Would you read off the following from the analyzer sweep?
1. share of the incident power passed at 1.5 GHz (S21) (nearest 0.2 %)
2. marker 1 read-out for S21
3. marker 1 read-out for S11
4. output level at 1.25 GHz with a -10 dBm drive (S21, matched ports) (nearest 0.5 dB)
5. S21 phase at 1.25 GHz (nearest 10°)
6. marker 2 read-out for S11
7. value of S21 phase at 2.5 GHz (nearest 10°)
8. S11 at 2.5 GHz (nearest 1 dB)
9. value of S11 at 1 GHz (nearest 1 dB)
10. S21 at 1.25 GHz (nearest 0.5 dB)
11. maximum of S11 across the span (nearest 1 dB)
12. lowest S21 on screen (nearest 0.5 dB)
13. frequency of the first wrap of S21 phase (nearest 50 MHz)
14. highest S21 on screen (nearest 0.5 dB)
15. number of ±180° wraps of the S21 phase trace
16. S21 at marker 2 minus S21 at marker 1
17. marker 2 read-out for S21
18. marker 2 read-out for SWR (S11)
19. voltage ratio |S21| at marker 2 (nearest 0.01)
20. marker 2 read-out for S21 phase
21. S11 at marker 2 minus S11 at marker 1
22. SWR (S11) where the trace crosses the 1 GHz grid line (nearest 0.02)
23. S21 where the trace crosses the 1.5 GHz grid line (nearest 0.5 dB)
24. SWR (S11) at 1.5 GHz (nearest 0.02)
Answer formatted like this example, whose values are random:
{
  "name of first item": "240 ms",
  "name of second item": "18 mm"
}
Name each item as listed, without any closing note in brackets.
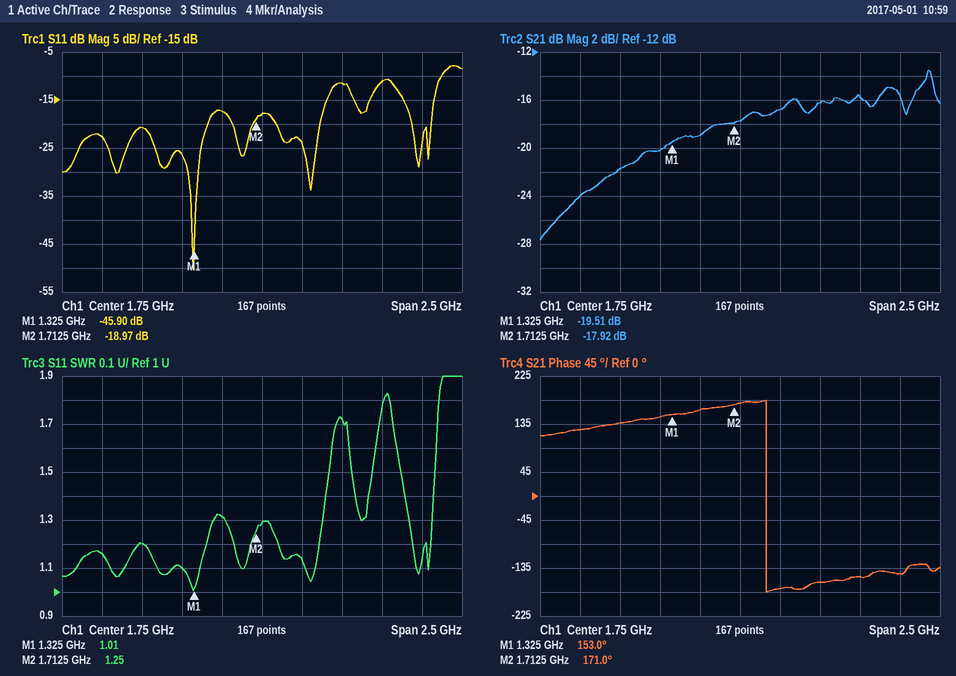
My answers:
{
  "share of the incident power passed at 1.5 GHz (S21)": "1.2 %",
  "marker 1 read-out for S21": "-19.51 dB",
  "marker 1 read-out for S11": "-45.90 dB",
  "output level at 1.25 GHz with a -10 dBm drive (S21, matched ports)": "-30.0 dBm",
  "S21 phase at 1.25 GHz": "150°",
  "marker 2 read-out for S11": "-18.97 dB",
  "value of S21 phase at 2.5 GHz": "-150°",
  "S11 at 2.5 GHz": "-11 dB",
  "value of S11 at 1 GHz": "-21 dB",
  "S21 at 1.25 GHz": "-20.0 dB",
  "maximum of S11 across the span": "-8 dB",
  "lowest S21 on screen": "-27.5 dB",
  "frequency of the first wrap of S21 phase": "1.90 GHz",
  "highest S21 on screen": "-13.5 dB",
  "number of ±180° wraps of the S21 phase trace": "1",
  "S21 at marker 2 minus S21 at marker 1": "1.59 dB",
  "marker 2 read-out for S21": "-17.92 dB",
  "marker 2 read-out for SWR": "1.25",
  "voltage ratio |S21| at marker 2": "0.13",
  "marker 2 read-out for S21 phase": "171.0°",
  "S11 at marker 2 minus S11 at marker 1": "26.93 dB",
  "SWR (S11) where the trace crosses the 1 GHz grid line": "1.20",
  "S21 where the trace crosses the 1.5 GHz grid line": "-19.0 dB",
  "SWR (S11) at 1.5 GHz": "1.32"
}
